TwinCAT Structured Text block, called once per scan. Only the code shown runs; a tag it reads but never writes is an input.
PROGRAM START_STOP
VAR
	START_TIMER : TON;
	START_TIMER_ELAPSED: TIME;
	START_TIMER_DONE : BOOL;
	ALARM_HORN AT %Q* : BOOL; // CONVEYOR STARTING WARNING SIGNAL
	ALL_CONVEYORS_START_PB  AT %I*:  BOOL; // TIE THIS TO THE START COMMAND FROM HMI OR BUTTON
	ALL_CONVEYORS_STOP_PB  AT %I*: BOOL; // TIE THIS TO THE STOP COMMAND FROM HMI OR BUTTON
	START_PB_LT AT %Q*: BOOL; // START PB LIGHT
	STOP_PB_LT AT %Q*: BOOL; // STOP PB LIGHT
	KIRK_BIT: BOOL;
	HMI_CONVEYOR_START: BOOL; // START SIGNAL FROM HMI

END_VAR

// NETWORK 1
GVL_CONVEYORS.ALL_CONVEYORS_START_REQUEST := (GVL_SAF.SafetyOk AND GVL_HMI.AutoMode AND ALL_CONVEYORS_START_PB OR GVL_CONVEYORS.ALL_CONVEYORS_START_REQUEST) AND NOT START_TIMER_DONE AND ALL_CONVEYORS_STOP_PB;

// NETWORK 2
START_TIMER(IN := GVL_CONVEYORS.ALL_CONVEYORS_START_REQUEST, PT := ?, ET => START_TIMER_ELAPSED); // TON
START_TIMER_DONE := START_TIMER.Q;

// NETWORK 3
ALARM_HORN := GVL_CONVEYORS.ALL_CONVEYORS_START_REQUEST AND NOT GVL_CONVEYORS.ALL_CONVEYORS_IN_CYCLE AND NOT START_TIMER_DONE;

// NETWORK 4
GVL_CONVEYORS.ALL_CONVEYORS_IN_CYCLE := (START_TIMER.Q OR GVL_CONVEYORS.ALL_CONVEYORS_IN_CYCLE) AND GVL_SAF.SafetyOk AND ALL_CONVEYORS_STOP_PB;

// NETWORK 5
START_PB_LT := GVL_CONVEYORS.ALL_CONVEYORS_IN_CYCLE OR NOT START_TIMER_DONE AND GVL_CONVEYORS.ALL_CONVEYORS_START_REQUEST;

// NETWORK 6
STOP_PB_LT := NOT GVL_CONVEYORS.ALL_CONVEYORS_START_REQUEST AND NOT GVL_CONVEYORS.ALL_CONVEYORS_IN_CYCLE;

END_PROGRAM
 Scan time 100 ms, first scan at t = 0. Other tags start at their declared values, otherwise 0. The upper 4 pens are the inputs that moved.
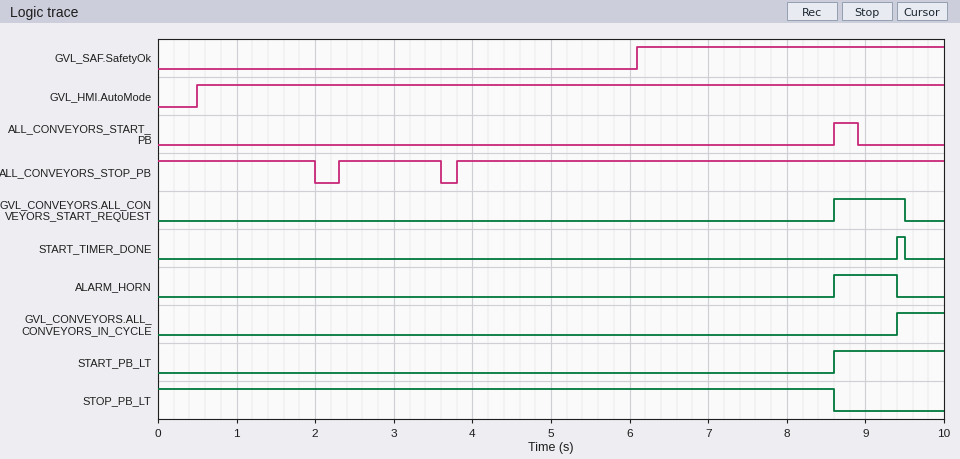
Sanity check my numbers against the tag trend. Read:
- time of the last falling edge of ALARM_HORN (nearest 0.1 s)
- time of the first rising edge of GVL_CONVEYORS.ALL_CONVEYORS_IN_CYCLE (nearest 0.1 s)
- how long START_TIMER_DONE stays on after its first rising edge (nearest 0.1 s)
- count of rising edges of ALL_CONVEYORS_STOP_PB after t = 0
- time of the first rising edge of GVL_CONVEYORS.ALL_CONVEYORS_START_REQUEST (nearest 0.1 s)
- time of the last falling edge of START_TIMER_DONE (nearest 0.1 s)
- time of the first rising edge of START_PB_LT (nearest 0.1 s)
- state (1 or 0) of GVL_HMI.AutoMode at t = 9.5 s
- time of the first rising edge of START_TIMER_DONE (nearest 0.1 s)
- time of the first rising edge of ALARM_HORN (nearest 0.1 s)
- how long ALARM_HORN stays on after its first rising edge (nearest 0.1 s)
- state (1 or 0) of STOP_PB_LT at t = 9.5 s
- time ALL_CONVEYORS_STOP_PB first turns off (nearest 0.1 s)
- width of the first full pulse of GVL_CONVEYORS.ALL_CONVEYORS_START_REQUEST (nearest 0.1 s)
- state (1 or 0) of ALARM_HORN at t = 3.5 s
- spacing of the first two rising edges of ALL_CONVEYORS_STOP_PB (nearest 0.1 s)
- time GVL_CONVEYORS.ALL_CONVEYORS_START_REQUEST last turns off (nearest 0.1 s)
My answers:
9.4 s
9.4 s
0.1 s
2
8.6 s
9.5 s
8.6 s
1
9.4 s
8.6 s
0.8 s
0
2.0 s
0.9 s
0
1.5 s
9.5 s
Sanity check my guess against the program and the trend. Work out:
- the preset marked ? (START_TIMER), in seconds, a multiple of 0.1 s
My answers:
0.8 s
